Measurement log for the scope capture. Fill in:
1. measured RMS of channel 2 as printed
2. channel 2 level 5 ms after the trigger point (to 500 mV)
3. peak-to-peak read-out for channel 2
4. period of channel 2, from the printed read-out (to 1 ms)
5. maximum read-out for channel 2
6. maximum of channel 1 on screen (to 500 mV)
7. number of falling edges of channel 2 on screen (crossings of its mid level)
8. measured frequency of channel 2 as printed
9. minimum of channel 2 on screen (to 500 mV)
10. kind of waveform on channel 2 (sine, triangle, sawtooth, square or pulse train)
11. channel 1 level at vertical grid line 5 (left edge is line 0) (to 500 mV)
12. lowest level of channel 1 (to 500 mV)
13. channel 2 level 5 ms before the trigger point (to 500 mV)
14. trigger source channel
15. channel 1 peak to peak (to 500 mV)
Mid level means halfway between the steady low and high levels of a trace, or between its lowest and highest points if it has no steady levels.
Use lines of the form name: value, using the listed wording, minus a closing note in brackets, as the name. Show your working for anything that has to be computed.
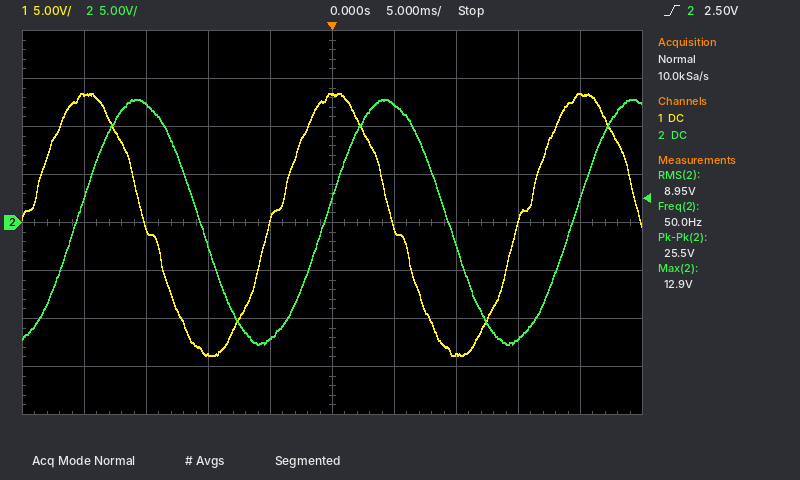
measured RMS of channel 2 as printed: 8.95 V
channel 2 level 5 ms after the trigger point: 12.5 V
peak-to-peak read-out for channel 2: 25.5 V
period of channel 2, from the printed read-out: 1 / 50.0 Hz ≈ 20 ms
maximum read-out for channel 2: 12.9 V
maximum of channel 1 on screen: 13.5 V
number of falling edges of channel 2 on screen: 2
measured frequency of channel 2 as printed: 50.0 Hz
minimum of channel 2 on screen: -12.5 V
kind of waveform on channel 2: sine
channel 1 level at vertical grid line 5 (left edge is line 0): 13.5 V
lowest level of channel 1: -14.0 V
channel 2 level 5 ms before the trigger point: -12.0 V
trigger source channel: channel 2
channel 1 peak to peak: 13.5 V − (-14.0 V) = 27.5 V
